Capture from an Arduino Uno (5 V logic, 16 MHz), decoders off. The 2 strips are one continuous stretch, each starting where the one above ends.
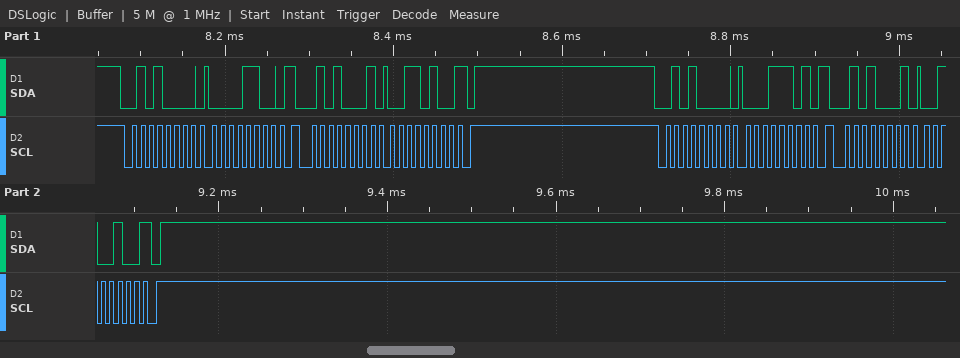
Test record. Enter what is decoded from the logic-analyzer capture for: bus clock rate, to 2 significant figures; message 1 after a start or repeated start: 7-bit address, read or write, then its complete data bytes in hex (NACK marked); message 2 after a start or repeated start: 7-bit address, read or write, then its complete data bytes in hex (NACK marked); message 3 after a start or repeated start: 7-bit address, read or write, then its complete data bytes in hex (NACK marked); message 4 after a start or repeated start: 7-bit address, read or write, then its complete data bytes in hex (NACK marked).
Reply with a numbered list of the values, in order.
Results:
1. 100 kHz
2. 0x28 write: 0C
3. 0x28 read: 34 NACK
4. 0x28 write: 1D
5. 0x28 read: 24 NACK
